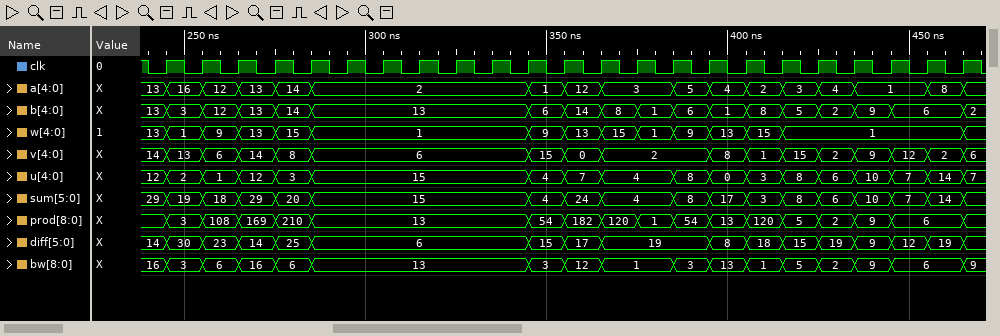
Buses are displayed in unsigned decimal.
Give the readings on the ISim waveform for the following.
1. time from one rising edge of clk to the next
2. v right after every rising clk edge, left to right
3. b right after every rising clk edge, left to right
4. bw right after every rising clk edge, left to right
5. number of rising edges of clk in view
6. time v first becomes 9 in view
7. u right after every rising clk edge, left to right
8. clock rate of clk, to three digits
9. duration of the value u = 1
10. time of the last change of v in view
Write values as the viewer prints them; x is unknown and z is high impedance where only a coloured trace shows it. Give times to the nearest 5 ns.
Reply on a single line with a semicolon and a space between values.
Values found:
10 ns; 13, 6, 14, 8, 6, 6, 6, 6, 6, 6, 15, 0, 2, 2, 2, 8, 1, 15, 2, 9, 12, 2, 6; 3, 12, 13, 14, 13, 13, 13, 13, 13, 13, 6, 14, 8, 1, 6, 1, 8, 5, 2, 9, 6, 6, 2; 3, 6, 16, 6, 13, 13, 13, 13, 13, 13, 3, 12, 1, 1, 3, 13, 1, 5, 2, 9, 6, 6, 9; 23; 435 ns; 2, 1, 12, 3, 15, 15, 15, 15, 15, 15, 4, 7, 4, 4, 8, 0, 3, 8, 6, 10, 7, 14, 7; 100 MHz; 10 ns; 465 ns
